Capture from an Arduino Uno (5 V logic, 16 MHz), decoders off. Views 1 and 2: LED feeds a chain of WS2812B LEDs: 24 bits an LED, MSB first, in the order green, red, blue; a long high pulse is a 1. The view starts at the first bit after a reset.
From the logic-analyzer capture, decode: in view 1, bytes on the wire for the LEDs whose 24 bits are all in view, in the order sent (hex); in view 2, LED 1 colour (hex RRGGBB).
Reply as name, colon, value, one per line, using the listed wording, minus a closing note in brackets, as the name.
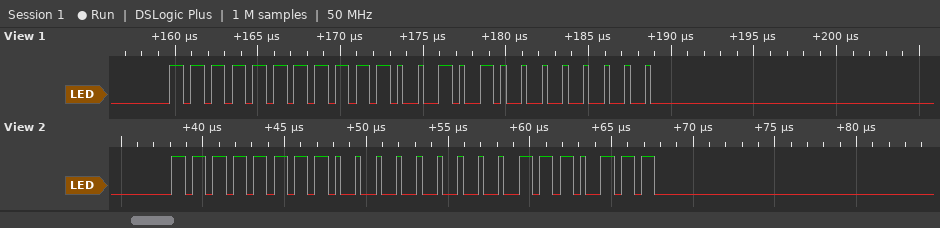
in view 1, bytes on the wire for the LEDs whose 24 bits are all in view, in the order sent: FF E5 00
in view 2, LED 1 colour: #00FF77
